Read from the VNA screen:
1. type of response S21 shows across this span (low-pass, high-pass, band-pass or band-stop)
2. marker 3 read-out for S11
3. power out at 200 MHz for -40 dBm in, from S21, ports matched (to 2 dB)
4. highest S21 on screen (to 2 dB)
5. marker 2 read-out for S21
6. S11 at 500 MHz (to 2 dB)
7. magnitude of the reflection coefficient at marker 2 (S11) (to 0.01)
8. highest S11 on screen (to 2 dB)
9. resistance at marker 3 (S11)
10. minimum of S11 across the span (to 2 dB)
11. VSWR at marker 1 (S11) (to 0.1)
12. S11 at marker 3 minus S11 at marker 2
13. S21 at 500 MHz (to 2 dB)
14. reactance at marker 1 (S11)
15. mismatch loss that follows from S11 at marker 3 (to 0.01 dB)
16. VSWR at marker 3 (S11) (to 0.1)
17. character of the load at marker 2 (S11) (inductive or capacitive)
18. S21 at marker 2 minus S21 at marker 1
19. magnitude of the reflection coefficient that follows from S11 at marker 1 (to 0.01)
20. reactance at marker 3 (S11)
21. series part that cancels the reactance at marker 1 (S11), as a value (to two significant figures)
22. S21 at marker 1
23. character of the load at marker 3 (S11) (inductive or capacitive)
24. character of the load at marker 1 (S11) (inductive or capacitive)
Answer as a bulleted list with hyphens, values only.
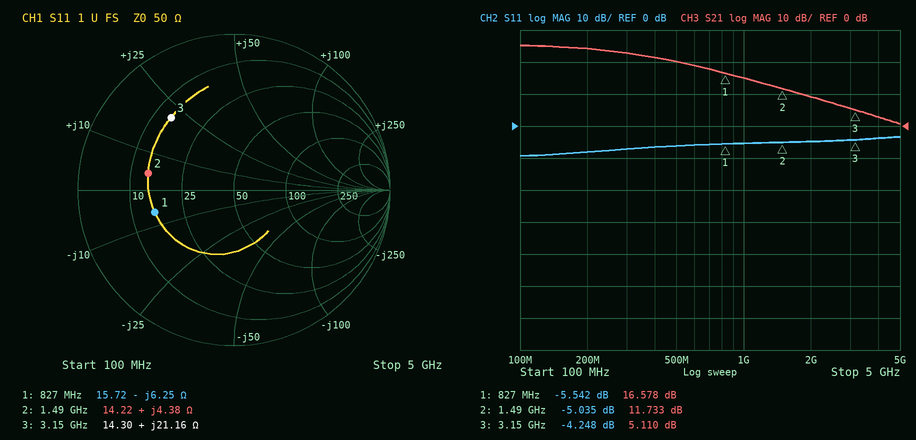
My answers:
- low-pass
- -4.248 dB
- -16 dBm
- 26 dB
- 11.733 dB
- -6 dB
- 0.56
- -4 dB
- 14.30 Ω
- -10 dB
- 3.2
- 0.787 dB
- 20 dB
- -6.25 Ω
- 2.05 dB
- 4.2
- inductive
- -4.845 dB
- 0.53
- +21.16 Ω
- 1.2 nH
- 16.578 dB
- inductive
- capacitive
